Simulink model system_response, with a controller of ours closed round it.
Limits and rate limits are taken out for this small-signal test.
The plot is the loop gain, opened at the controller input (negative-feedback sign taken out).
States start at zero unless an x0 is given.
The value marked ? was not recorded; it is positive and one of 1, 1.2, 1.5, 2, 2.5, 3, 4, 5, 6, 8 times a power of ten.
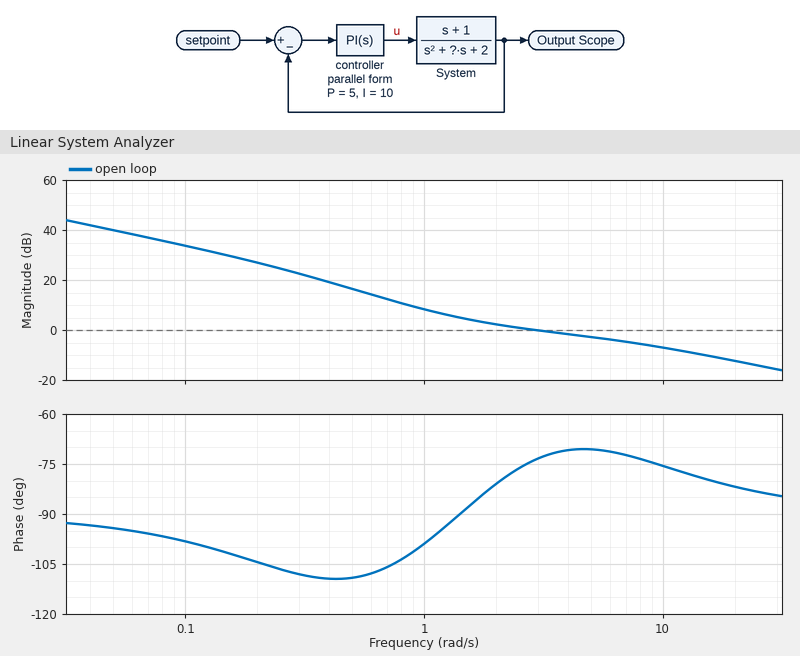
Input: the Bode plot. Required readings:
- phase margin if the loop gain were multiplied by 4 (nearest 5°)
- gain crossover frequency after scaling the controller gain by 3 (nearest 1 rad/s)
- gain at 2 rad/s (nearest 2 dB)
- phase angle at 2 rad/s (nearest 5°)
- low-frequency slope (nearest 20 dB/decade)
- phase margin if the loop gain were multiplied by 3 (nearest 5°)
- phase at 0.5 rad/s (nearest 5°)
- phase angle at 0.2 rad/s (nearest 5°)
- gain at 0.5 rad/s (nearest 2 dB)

100°
14 rad/s
2 dB
-80°
-20 dB/decade
100°
-110°
-105°
16 dB
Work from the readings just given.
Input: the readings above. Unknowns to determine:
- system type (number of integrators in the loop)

1
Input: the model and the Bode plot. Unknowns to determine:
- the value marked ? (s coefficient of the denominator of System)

6
